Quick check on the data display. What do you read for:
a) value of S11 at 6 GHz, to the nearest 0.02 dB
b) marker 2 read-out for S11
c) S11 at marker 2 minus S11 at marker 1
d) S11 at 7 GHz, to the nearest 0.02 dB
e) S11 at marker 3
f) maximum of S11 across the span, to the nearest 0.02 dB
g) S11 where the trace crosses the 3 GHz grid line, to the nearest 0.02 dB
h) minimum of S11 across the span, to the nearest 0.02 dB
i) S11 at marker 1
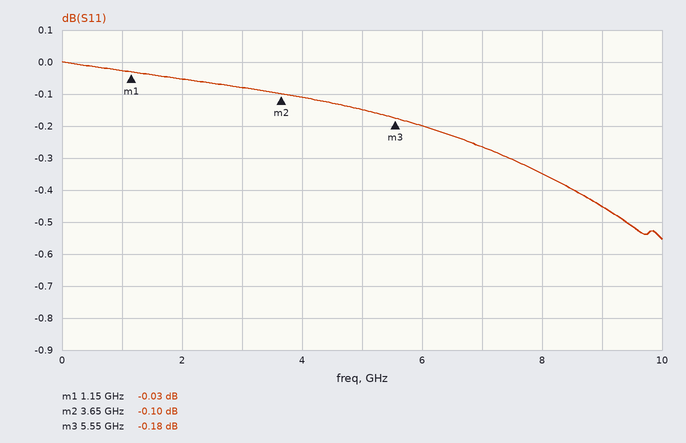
-0.20 dB
-0.10 dB
-0.07 dB
-0.26 dB
-0.18 dB
0.00 dB
-0.08 dB
-0.56 dB
-0.03 dB
